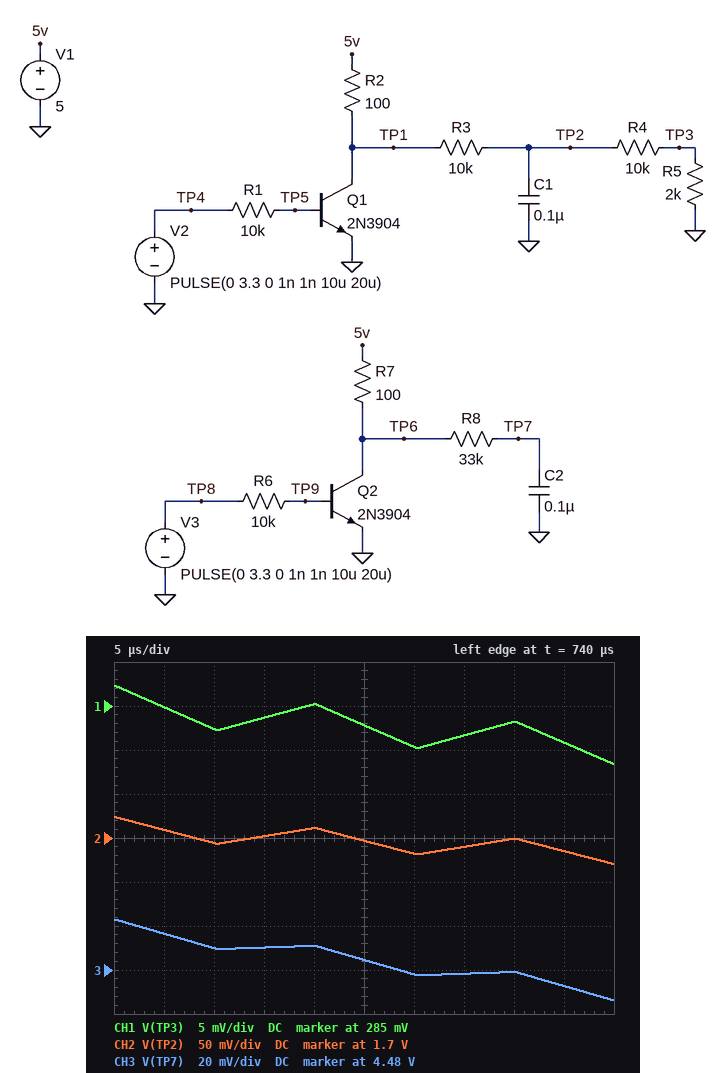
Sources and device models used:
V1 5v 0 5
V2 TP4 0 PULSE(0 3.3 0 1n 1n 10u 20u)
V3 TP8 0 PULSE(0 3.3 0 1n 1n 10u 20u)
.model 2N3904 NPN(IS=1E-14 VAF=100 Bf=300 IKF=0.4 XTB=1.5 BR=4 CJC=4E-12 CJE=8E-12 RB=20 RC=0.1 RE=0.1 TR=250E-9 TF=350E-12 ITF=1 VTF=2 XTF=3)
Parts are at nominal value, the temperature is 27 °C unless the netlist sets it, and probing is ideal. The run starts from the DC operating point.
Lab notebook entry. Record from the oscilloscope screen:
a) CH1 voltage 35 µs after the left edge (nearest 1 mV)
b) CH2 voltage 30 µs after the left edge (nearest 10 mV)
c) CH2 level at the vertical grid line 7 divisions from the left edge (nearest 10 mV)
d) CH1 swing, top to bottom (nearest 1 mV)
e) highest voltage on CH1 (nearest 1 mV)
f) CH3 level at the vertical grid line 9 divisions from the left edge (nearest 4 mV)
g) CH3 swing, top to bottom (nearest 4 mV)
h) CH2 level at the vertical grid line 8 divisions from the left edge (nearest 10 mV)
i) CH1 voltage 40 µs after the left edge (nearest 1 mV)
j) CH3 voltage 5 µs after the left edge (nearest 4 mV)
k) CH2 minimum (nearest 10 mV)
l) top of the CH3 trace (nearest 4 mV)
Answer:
282 mV
1.68 V
1.69 V
9 mV
287 mV
4.472 V
36 mV
1.70 V
283 mV
4.496 V
1.67 V
4.504 V
